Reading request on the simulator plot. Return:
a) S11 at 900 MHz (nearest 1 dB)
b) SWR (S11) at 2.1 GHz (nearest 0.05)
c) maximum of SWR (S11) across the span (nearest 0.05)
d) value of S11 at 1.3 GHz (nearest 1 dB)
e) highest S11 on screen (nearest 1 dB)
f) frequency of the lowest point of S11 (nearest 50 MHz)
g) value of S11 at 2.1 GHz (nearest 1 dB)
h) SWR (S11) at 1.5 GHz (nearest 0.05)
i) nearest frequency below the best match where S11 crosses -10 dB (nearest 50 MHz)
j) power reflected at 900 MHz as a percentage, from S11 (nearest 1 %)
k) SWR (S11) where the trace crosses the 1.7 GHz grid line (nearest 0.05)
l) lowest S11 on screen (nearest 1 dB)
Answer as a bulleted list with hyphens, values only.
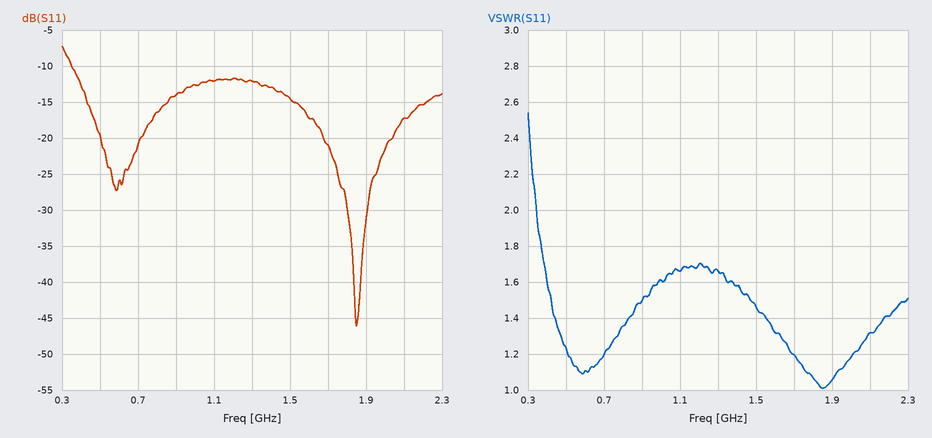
- -14 dB
- 1.30
- 2.55
- -12 dB
- -7 dB
- 1.85 GHz
- -17 dB
- 1.45
- 350 MHz
- 4 %
- 1.20
- -46 dB
